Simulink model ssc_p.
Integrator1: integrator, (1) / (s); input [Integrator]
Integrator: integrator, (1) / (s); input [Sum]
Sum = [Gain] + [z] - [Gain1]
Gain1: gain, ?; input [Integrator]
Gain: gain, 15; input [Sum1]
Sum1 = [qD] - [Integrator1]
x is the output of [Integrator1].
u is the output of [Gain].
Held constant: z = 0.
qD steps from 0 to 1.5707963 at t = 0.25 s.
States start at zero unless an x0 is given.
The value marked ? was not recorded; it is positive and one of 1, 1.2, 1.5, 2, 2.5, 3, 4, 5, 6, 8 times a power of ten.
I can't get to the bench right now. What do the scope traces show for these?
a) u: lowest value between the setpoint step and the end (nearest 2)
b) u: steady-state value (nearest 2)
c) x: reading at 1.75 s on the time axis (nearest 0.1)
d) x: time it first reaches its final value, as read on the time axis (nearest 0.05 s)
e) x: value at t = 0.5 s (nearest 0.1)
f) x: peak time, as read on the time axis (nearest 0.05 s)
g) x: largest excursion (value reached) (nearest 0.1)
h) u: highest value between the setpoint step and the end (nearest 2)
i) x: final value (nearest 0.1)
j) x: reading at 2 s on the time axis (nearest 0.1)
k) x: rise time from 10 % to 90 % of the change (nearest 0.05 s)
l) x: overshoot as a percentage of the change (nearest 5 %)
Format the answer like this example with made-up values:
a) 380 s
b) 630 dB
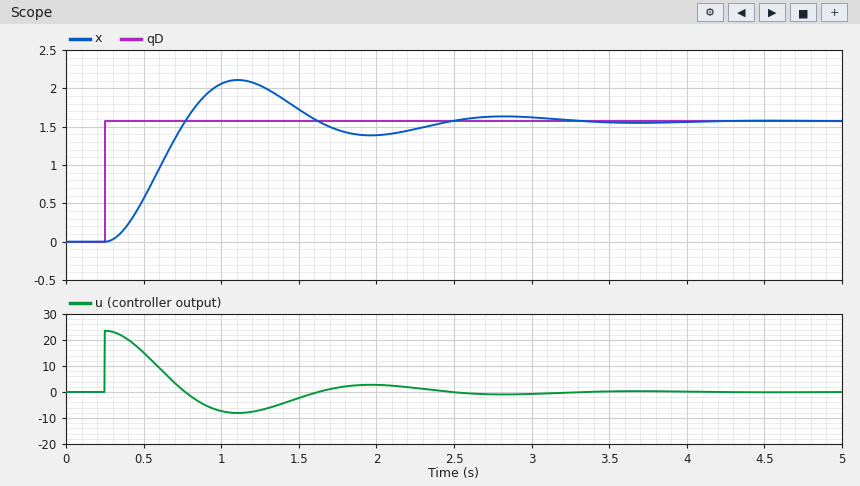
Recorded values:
a) -8
b) 0
c) 1.5
d) 0.75 s
e) 0.6
f) 1.10 s
g) 2.1
h) 24
i) 1.6
j) 1.4
k) 0.35 s
l) 35 %
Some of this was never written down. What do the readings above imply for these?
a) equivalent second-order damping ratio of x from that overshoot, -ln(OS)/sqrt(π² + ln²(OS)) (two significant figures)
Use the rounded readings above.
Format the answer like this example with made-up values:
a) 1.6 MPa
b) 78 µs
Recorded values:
a) 0.32
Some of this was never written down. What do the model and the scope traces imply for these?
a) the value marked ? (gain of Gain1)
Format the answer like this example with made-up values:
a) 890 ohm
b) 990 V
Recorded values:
a) 2.5
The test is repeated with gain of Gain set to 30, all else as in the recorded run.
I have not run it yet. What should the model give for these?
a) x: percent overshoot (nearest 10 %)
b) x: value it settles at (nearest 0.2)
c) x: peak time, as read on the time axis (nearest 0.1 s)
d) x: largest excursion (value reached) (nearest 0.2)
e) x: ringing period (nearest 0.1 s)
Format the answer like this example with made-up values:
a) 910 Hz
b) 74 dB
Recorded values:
a) 50 %
b) 1.6
c) 0.8 s
d) 2.4
e) 1.2 s
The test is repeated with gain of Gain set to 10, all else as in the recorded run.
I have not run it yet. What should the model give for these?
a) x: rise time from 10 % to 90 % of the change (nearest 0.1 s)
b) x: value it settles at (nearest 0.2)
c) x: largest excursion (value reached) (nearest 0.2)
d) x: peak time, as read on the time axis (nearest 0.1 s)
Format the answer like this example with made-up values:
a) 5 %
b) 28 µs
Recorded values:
a) 0.5 s
b) 1.6
c) 2.0
d) 1.3 s
